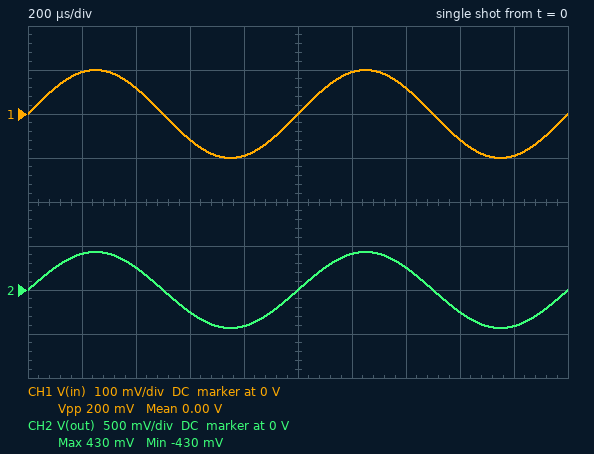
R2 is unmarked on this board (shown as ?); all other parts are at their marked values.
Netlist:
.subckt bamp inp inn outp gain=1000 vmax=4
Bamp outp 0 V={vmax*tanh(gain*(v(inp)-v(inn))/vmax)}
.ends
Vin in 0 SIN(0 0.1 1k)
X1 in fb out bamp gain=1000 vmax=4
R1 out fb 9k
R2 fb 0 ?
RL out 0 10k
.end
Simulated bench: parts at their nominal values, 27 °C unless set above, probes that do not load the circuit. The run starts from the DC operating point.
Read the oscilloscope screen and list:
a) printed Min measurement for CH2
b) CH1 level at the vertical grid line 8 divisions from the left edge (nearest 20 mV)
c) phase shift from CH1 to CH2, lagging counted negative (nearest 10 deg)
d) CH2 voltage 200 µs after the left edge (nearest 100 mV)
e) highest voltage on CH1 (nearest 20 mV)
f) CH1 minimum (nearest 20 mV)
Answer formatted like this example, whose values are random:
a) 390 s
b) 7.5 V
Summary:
a) -430 mV
b) -60 mV
c) 0 deg
d) 400 mV
e) 100 mV
f) -100 mV
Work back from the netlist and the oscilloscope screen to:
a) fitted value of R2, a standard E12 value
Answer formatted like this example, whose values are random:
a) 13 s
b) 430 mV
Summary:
a) 2.7 kΩ
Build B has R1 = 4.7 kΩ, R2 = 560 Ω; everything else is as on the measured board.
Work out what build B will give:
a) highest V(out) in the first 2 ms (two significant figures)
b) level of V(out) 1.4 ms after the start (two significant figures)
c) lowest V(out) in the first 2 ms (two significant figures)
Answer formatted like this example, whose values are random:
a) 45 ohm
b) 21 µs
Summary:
a) 930 mV
b) 550 mV
c) -930 mV
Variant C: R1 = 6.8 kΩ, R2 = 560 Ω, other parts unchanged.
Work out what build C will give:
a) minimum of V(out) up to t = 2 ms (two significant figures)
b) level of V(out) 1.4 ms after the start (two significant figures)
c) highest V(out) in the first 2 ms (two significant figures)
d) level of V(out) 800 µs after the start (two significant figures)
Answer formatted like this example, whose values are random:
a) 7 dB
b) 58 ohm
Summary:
a) -1.3 V
b) 760 mV
c) 1.3 V
d) -1.2 V
